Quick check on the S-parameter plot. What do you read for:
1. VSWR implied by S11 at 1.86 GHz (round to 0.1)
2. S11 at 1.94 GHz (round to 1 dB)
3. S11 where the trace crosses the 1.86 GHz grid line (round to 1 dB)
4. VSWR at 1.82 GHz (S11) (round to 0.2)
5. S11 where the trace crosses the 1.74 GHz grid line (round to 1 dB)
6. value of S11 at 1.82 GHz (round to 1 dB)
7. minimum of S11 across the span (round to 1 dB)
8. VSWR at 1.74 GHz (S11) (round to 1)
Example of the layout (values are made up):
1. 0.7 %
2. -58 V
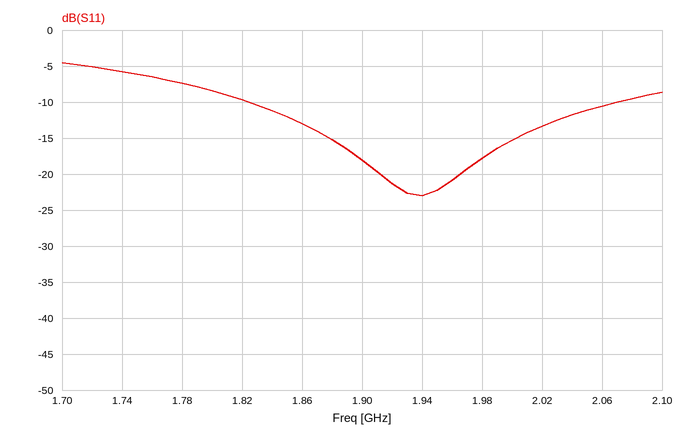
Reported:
1. 1.6
2. -23 dB
3. -13 dB
4. 2.0
5. -6 dB
6. -10 dB
7. -23 dB
8. 3
